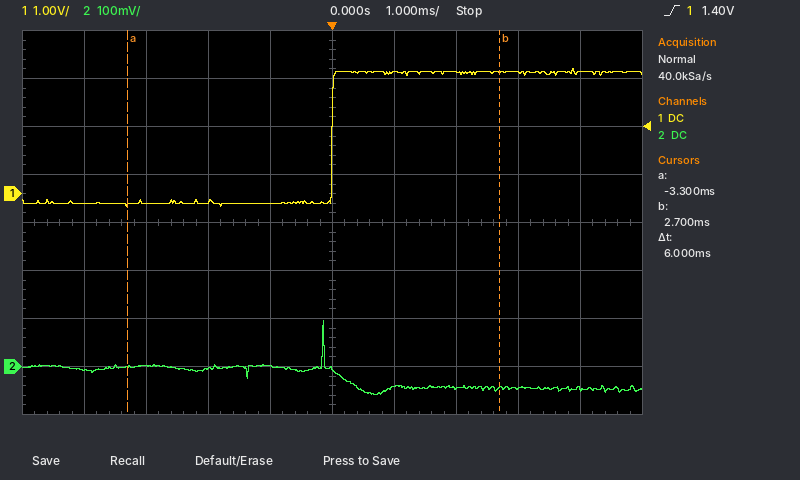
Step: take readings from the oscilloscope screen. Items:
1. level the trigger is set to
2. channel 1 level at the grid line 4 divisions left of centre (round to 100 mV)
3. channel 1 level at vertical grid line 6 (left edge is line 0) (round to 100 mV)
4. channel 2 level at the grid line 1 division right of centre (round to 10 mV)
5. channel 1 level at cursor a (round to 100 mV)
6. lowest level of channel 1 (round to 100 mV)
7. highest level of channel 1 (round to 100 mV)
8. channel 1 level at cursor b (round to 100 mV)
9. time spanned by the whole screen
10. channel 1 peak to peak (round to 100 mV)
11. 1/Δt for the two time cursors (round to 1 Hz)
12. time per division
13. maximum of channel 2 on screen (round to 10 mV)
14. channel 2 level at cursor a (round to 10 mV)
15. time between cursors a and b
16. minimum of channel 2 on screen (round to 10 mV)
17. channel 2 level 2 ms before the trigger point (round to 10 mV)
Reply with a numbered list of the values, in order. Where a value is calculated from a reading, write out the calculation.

1. 1.40 V
2. -200 mV
3. 2.5 V
4. -40 mV
5. -200 mV
6. -300 mV
7. 2.6 V
8. 2.5 V
9. 10 ms
10. 2.6 V − (-300 mV) = 2.9 V
11. 1 / 6 ms ≈ 167 Hz
12. 1 ms
13. 100 mV
14. 0 mV
15. 6 ms
16. -60 mV
17. 0 mV
